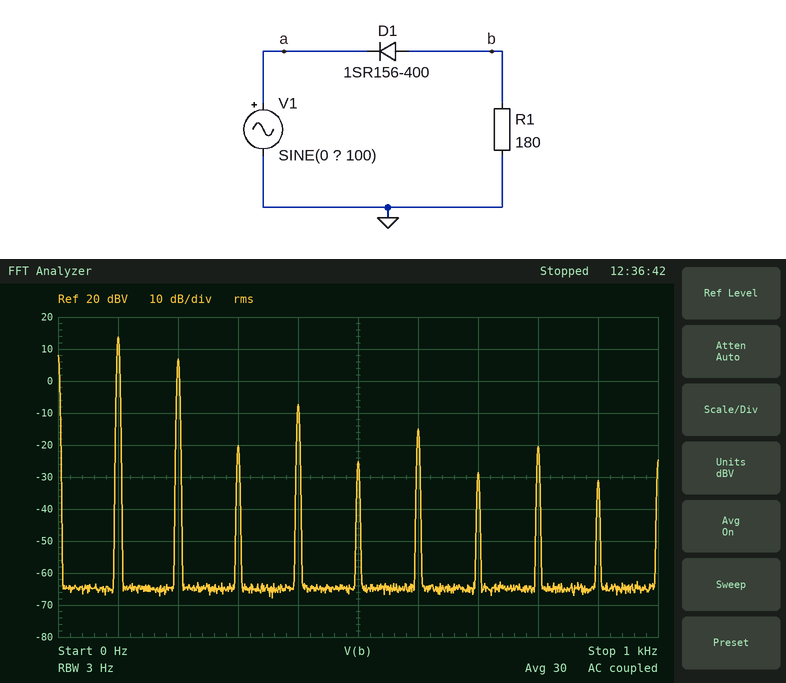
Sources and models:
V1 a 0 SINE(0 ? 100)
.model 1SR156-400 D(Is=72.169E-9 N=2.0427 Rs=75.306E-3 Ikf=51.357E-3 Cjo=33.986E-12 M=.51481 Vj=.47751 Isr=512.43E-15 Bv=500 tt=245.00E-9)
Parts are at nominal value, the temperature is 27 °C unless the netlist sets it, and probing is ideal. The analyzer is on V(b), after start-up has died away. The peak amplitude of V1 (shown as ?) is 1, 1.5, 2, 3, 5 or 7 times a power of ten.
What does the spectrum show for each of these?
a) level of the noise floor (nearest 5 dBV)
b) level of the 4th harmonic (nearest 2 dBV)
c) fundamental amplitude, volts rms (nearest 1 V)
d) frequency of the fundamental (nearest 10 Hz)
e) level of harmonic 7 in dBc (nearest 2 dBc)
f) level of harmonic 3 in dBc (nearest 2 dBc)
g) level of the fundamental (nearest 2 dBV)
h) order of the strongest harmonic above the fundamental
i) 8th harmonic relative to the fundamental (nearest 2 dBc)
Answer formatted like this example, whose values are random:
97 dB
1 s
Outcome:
-65 dBV
-8 dBV
5 V
100 Hz
-42 dBc
-34 dBc
14 dBV
2
-34 dBc
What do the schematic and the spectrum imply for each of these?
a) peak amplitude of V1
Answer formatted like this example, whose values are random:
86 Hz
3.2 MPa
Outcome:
15 V
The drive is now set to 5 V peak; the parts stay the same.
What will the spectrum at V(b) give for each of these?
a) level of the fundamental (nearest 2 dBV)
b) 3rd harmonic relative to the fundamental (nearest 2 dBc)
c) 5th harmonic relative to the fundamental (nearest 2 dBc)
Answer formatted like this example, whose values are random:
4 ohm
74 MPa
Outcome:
4 dBV
-24 dBc
-30 dBc
